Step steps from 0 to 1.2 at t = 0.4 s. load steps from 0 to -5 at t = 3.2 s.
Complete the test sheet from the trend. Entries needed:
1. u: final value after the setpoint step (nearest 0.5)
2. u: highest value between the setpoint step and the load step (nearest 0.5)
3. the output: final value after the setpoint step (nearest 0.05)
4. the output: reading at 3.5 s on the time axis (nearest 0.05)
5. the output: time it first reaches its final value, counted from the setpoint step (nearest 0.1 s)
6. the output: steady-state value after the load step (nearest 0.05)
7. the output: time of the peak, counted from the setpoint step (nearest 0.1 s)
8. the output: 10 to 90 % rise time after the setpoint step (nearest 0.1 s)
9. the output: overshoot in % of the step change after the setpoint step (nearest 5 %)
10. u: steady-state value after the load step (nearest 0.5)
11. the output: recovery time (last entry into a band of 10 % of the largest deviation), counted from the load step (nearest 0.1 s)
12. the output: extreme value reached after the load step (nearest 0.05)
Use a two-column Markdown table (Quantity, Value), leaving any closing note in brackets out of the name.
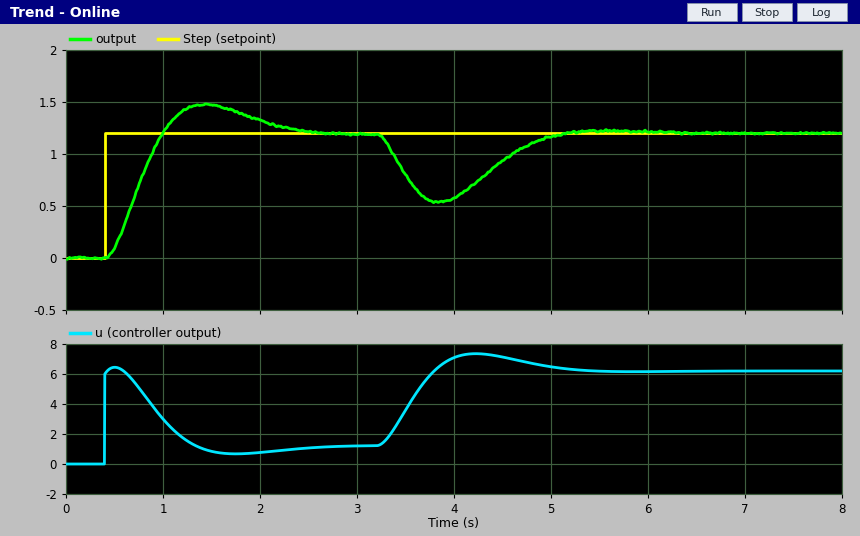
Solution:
| Quantity | Value |
|---|---|
| u: final value after the setpoint step | 1.0 |
| u: highest value between the setpoint step and the load step | 6.5 |
| the output: final value after the setpoint step | 1.20 |
| the output: reading at 3.5 s on the time axis | 0.80 |
| the output: time it first reaches its final value, counted from the setpoint step | 0.6 s |
| the output: steady-state value after the load step | 1.20 |
| the output: time of the peak, counted from the setpoint step | 1.0 s |
| the output: 10 to 90 % rise time after the setpoint step | 0.4 s |
| the output: overshoot in % of the step change after the setpoint step | 25 % |
| u: steady-state value after the load step | 6.0 |
| the output: recovery time (last entry into a band of 10 % of the largest deviation), counted from the load step | 1.7 s |
| the output: extreme value reached after the load step | 0.55 |
